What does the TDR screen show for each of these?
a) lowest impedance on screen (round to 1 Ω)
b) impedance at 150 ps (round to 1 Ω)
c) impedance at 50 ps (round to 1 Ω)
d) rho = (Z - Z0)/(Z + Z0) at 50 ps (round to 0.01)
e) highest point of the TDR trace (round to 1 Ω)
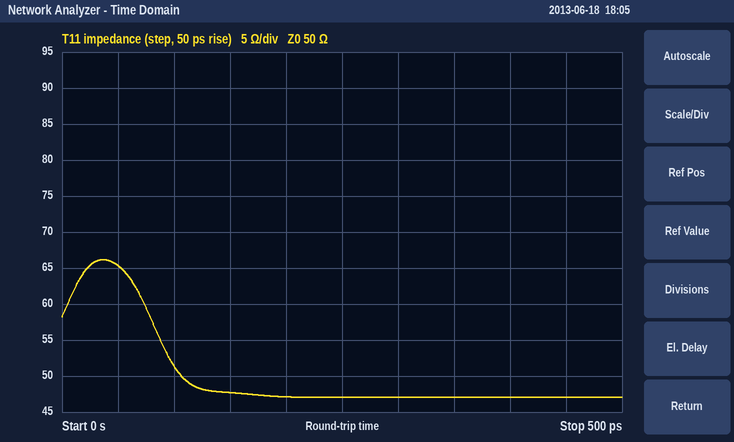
47 Ω
48 Ω
65 Ω
+0.13
66 Ω
